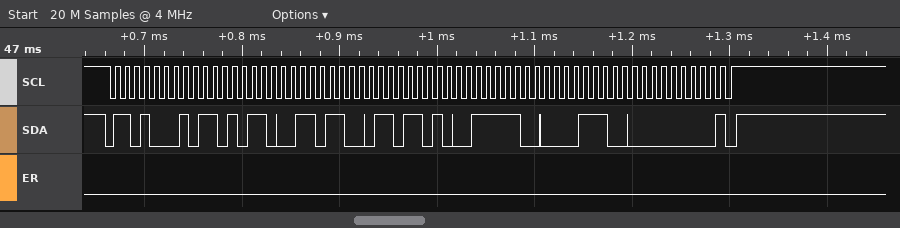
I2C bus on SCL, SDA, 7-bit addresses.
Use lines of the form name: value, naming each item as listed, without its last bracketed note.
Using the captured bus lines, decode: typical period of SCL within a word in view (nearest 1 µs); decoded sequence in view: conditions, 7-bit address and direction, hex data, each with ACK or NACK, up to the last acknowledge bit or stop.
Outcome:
typical period of SCL within a word in view: 10 µs
decoded sequence in view: conditions, 7-bit address and direction, hex data, each with ACK or NACK, up to the last acknowledge bit or stop: start, address 68 read ACK, D6 ACK, 6C ACK, DA ACK, 7C ACK, 1C ACK, 00 NACK, stop
